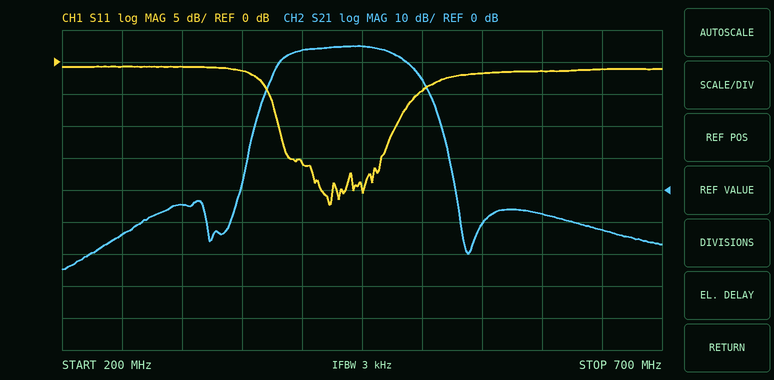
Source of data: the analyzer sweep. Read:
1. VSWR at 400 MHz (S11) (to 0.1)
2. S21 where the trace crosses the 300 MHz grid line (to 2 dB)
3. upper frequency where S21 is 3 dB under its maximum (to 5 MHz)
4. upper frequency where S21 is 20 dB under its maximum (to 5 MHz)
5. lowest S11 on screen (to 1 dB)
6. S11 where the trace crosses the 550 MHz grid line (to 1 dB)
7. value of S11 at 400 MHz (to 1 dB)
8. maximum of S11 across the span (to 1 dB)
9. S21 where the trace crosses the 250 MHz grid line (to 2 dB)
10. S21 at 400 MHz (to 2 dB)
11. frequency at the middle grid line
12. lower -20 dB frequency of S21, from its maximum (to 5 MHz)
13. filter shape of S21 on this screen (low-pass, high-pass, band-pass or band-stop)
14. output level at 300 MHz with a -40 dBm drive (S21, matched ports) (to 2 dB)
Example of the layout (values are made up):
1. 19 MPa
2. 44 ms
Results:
1. 1.4
2. -4 dB
3. 480 MHz
4. 510 MHz
5. -22 dB
6. -2 dB
7. -16 dB
8. -1 dB
9. -14 dB
10. 44 dB
11. 450 MHz
12. 365 MHz
13. band-pass
14. -44 dBm
